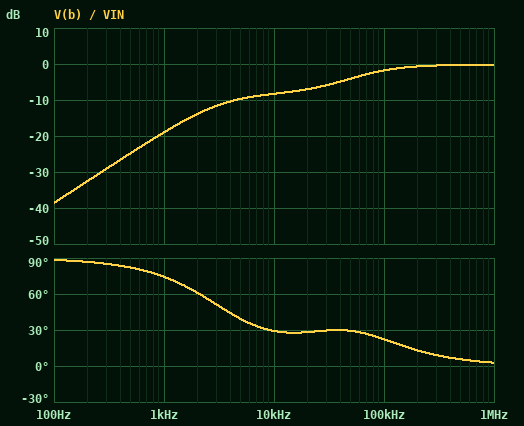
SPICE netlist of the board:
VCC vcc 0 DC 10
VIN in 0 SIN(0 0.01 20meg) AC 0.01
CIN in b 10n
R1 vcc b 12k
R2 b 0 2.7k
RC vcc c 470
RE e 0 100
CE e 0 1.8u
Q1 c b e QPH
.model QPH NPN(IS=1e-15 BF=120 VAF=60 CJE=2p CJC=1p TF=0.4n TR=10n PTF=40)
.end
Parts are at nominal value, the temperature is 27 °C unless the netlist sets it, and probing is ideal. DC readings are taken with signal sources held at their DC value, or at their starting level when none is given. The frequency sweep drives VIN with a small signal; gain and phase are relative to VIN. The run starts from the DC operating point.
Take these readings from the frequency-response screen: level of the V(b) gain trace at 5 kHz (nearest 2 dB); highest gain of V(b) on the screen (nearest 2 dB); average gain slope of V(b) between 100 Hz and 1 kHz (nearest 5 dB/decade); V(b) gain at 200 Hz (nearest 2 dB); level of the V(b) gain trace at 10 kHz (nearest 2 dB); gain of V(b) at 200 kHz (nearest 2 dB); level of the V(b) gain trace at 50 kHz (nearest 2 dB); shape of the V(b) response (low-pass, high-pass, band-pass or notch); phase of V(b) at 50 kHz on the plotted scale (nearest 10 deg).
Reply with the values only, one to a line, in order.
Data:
-10 dB
0 dB
20 dB/decade
-32 dB
-8 dB
0 dB
-4 dB
high-pass
30 deg
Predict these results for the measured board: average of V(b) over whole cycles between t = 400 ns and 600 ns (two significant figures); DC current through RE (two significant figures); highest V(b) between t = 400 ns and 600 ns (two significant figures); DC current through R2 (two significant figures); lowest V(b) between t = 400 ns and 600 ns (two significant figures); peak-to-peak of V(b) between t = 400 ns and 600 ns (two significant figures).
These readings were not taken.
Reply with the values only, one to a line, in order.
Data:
1.7 V
9.1 mA
1.7 V
620 µA
1.7 V
20 mV
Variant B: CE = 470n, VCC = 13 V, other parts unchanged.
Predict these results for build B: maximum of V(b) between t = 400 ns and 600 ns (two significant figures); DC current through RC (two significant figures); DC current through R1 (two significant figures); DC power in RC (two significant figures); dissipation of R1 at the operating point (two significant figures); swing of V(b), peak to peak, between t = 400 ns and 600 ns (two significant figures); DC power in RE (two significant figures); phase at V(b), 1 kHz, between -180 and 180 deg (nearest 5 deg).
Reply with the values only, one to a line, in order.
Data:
2.2 V
14 mA
900 µA
87 mW
9.8 mW
19 mV
19 mW
80 deg
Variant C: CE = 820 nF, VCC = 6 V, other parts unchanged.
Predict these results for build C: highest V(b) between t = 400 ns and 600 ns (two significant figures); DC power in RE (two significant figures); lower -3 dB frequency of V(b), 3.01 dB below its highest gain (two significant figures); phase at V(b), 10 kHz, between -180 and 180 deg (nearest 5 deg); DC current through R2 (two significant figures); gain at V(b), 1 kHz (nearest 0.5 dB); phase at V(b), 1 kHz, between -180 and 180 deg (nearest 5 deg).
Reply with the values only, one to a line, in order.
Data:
1.1 V
940 µW
24 kHz
35 deg
390 µA
-18.5 dB
80 deg
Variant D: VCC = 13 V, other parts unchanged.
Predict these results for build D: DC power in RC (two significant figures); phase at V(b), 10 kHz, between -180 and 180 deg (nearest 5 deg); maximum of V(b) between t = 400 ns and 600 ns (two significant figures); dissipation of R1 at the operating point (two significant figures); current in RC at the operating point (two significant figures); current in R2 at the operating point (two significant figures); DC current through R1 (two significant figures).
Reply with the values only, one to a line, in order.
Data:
87 mW
25 deg
2.2 V
9.8 mW
14 mA
800 µA
900 µA
